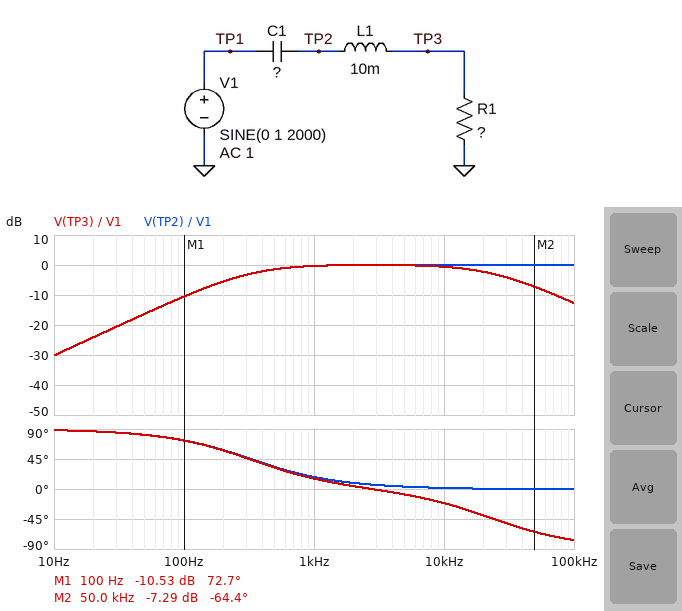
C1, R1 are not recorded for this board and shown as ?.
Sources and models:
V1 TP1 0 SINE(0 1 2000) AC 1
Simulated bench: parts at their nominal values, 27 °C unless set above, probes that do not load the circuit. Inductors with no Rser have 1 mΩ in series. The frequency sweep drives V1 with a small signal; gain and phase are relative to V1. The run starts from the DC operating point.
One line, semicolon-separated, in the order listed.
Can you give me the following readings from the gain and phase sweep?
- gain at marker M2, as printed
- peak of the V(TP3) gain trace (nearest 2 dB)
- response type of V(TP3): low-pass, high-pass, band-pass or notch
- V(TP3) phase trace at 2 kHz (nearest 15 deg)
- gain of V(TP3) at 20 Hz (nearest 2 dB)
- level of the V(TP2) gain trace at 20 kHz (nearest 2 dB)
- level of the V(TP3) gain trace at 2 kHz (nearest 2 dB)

-7.29 dB; 0 dB; band-pass; 0 deg; -24 dB; 0 dB; 0 dB
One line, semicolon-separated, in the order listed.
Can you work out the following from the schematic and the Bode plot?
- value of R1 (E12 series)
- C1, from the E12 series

1.5 kΩ; 330 nF
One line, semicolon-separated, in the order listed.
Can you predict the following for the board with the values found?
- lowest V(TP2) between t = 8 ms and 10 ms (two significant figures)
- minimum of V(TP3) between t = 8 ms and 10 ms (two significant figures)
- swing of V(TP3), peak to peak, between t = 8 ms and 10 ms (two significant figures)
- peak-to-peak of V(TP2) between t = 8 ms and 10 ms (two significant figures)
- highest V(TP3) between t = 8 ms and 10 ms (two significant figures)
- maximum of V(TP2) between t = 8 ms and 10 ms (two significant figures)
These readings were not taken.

-1.0 V; -1.0 V; 2.0 V; 2.0 V; 1.0 V; 1.0 V
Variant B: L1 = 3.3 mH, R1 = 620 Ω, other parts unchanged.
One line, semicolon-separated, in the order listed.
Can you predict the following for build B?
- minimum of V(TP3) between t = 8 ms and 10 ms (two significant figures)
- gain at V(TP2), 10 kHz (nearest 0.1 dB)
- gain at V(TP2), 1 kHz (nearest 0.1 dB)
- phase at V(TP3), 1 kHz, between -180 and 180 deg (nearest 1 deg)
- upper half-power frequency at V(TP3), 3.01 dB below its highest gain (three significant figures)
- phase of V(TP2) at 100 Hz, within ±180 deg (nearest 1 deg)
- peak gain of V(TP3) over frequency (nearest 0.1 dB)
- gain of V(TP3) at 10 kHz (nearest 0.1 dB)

-950 mV; 0.2 dB; -1.9 dB; 37 deg; 30.7 kHz; 83 deg; 0 dB; -0.3 dB
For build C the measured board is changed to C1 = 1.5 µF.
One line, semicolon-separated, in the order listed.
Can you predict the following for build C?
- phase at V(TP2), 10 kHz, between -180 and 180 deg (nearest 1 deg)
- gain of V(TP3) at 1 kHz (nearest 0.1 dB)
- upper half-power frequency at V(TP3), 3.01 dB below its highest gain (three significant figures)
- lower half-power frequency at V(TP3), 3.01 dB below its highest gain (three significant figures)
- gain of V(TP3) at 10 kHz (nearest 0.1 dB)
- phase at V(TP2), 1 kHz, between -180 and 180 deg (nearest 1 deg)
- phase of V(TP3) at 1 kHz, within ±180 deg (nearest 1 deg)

0 deg; 0 dB; 23.9 kHz; 70.5 Hz; -0.7 dB; 4 deg; 2 deg
